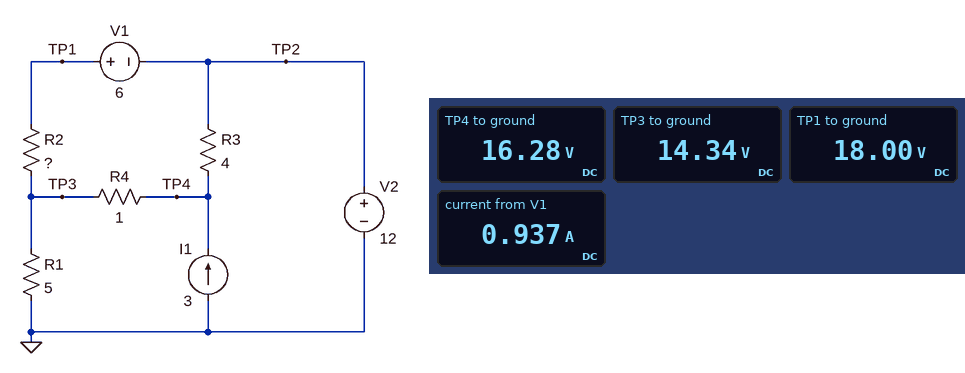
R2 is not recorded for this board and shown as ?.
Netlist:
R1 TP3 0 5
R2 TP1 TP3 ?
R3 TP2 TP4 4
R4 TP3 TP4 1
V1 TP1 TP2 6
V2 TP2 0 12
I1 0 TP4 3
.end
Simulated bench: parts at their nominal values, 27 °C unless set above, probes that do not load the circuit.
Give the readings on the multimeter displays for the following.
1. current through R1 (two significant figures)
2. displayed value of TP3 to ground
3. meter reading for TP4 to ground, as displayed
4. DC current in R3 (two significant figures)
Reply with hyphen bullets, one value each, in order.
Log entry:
- 2.9 A
- 14.34 V
- 16.28 V
- 1.1 A
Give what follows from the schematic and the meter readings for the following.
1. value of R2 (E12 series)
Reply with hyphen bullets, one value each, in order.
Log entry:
- 3.9 Ω
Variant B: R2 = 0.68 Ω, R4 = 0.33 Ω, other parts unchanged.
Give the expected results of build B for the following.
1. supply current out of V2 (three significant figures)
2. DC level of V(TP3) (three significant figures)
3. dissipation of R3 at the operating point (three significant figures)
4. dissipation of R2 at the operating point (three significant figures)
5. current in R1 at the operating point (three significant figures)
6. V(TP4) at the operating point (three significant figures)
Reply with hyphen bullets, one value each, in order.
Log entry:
- 367 mA
- 16.8 V
- 7.24 W
- 1.99 W
- 3.37 A
- 17.4 V
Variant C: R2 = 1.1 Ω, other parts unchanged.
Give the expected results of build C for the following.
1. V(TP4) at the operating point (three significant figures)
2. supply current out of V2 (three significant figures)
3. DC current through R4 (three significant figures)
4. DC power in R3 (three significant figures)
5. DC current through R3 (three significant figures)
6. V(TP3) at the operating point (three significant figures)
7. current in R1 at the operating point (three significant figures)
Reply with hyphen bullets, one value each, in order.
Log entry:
- 17.7 V
- 233 mA
- 1.57 A
- 8.22 W
- 1.43 A
- 16.2 V
- 3.23 A
